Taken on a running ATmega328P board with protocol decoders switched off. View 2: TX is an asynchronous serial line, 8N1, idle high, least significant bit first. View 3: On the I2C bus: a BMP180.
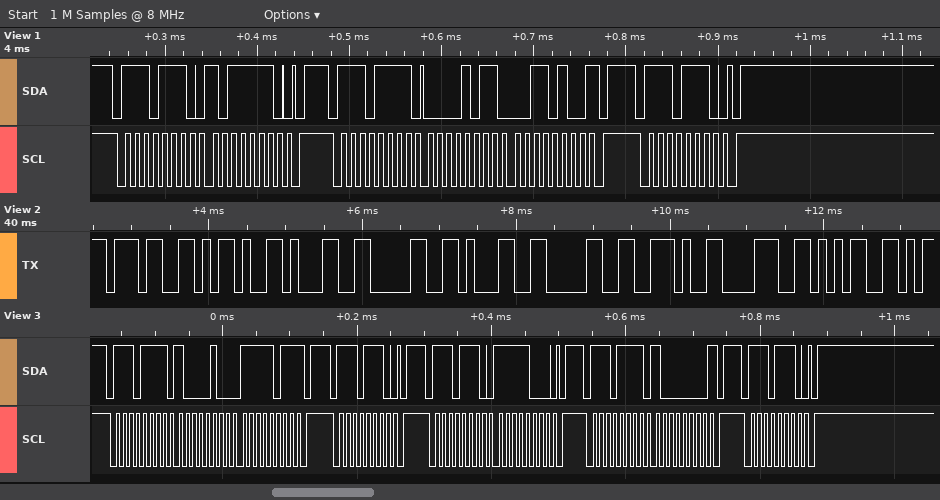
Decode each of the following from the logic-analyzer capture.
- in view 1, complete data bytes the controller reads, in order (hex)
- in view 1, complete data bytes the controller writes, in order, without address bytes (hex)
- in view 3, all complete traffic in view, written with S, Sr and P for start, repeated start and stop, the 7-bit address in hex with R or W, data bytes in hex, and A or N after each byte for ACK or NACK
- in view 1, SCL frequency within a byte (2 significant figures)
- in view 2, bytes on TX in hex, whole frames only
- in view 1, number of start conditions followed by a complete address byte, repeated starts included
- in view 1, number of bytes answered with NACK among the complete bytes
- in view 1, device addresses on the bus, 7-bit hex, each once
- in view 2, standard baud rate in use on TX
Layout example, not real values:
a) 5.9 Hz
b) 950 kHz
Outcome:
a) 0B 34
b) BE
c) S 77R A 84 A FB N P S 77W A P S 77W A F8 A P S 77R A 80 N P S 77W A P
d) 100 kHz
e) 37 2D 31 30 31 30 2E 38 35
f) 3
g) 1
h) 0x77
i) 9600 baud
